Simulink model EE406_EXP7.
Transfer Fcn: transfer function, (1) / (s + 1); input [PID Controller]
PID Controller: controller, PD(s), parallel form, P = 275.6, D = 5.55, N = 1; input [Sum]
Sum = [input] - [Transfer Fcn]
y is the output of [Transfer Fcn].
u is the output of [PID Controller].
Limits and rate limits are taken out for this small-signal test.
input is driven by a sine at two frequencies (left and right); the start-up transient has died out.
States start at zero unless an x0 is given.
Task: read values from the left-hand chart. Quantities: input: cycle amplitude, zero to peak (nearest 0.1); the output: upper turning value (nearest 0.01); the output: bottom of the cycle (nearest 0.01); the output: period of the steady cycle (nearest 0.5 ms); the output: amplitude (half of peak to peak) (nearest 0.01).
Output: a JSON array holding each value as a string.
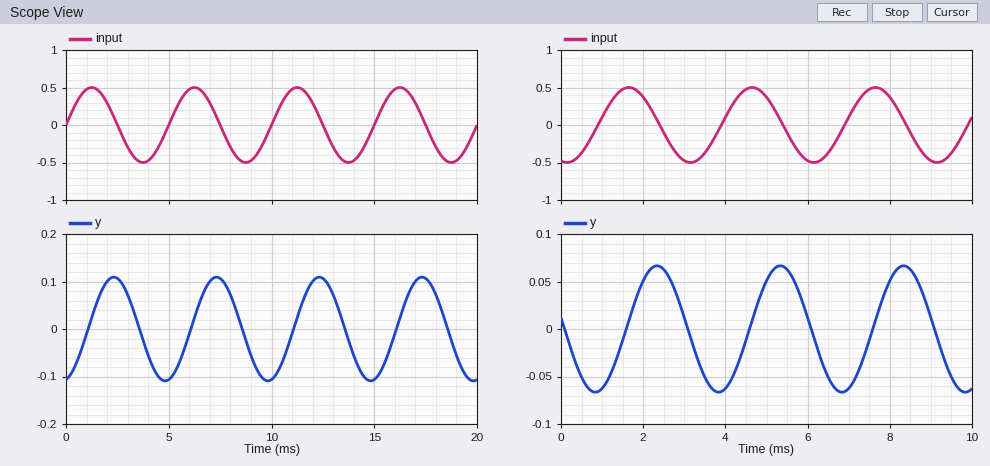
["0.5", "0.11", "-0.11", "5.0 ms", "0.11"]
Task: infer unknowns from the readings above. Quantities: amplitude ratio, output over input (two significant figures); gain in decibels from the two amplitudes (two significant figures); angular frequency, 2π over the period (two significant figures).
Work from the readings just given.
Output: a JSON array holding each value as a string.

["0.22", "-13 dB", "1.3 rad/ms"]
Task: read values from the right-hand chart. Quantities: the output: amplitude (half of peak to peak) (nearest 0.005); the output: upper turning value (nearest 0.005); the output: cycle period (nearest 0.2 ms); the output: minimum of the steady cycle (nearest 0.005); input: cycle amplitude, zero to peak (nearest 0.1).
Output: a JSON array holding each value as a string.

["0.065", "0.065", "3.0 ms", "-0.065", "0.5"]
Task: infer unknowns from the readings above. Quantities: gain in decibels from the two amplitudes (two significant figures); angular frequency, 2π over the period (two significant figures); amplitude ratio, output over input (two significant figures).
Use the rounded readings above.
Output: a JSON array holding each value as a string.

["-18 dB", "2.1 rad/ms", "0.13"]
